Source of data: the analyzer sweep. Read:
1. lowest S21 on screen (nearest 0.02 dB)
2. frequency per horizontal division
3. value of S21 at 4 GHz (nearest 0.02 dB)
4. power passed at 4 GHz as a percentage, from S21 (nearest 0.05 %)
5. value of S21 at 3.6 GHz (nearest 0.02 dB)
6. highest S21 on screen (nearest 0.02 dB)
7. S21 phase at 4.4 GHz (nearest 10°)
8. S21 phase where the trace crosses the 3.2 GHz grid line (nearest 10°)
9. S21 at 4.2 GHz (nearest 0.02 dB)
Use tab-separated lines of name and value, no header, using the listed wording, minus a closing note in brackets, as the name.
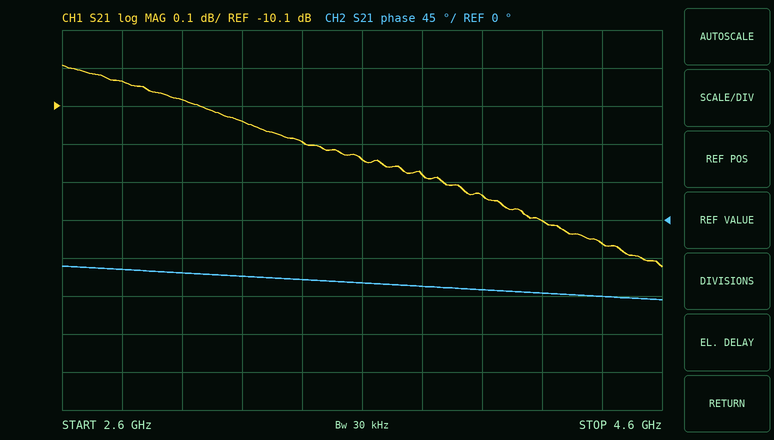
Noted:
lowest S21 on screen	-10.52 dB
frequency per horizontal division	200 MHz
value of S21 at 4 GHz	-10.34 dB
power passed at 4 GHz as a percentage, from S21	9.25 %
value of S21 at 3.6 GHz	-10.24 dB
highest S21 on screen	-10.00 dB
S21 phase at 4.4 GHz	-90°
S21 phase where the trace crosses the 3.2 GHz grid line	-70°
S21 at 4.2 GHz	-10.40 dB
